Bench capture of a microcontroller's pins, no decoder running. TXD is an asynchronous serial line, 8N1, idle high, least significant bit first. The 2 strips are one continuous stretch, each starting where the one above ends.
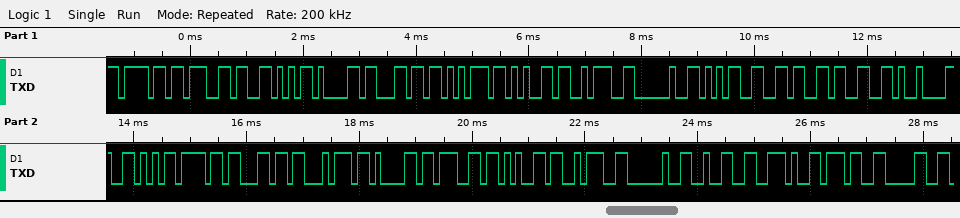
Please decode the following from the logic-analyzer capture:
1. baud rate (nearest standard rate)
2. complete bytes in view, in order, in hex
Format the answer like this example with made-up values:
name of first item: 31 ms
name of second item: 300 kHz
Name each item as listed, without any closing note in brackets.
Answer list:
baud rate: 9600 baud
complete bytes in view, in order, in hex: 6F 67 56 61 6C 75 65 3A 20 35 36 33 09 56 6F 6C 74 61 67 65 3A 20 32 2E 37 30
